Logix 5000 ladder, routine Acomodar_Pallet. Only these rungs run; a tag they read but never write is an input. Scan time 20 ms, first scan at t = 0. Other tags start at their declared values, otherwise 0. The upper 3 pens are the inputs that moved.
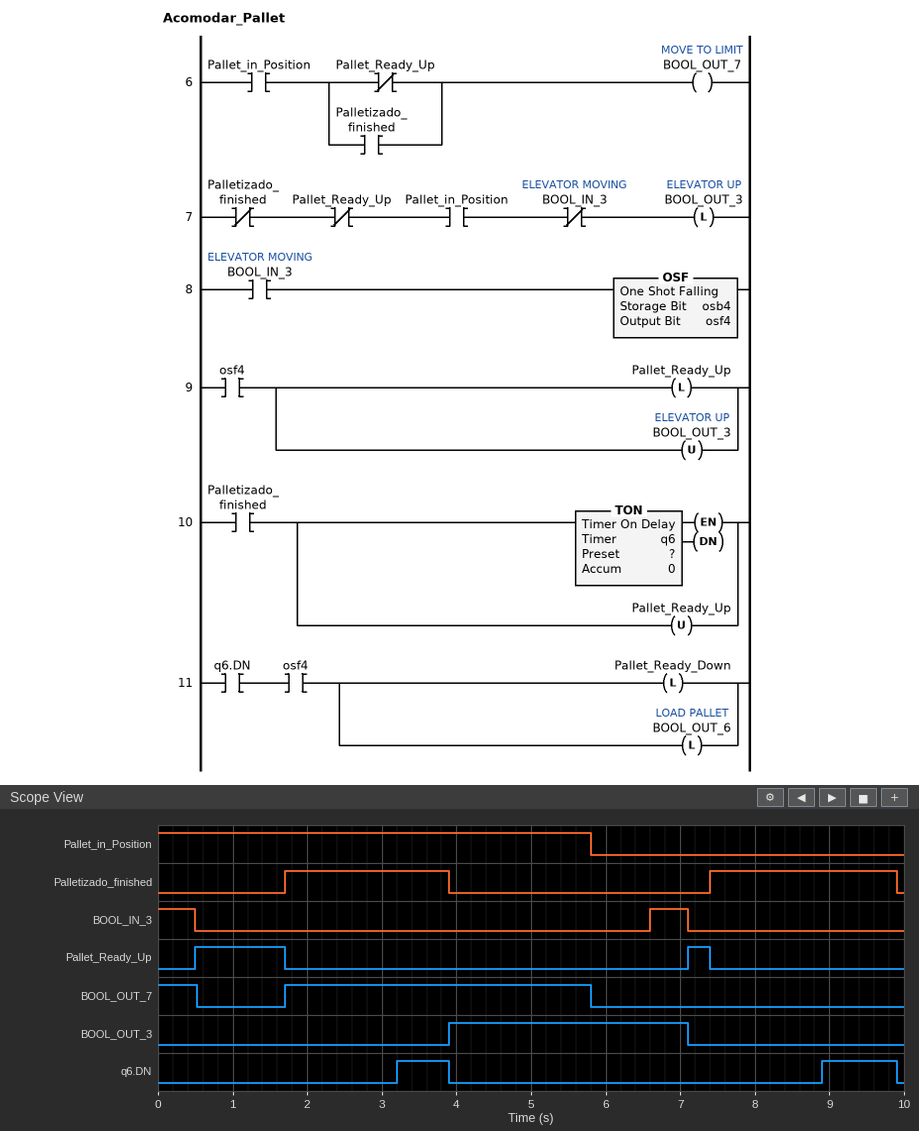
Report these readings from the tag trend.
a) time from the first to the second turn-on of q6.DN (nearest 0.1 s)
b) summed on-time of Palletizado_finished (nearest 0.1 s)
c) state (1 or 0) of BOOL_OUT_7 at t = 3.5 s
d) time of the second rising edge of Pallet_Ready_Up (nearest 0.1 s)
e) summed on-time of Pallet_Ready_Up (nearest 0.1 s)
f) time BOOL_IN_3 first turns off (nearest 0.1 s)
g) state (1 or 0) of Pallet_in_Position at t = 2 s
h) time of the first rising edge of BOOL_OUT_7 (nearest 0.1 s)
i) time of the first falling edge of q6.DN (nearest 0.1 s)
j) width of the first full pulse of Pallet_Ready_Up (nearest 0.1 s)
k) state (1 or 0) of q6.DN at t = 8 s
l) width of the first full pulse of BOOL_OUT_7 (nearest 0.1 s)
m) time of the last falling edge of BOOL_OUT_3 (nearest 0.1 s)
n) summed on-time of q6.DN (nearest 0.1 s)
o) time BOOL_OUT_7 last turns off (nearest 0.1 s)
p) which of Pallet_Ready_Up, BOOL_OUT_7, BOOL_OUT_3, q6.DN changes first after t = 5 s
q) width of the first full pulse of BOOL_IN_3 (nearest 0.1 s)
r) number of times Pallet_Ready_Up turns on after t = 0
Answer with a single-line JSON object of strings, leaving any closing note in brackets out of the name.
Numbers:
{"time from the first to the second turn-on of q6.DN": "5.7 s", "summed on-time of Palletizado_finished": "4.7 s", "state (1 or 0) of BOOL_OUT_7 at t = 3.5 s": "1", "time of the second rising edge of Pallet_Ready_Up": "7.1 s", "summed on-time of Pallet_Ready_Up": "1.5 s", "time BOOL_IN_3 first turns off": "0.5 s", "state (1 or 0) of Pallet_in_Position at t = 2 s": "1", "time of the first rising edge of BOOL_OUT_7": "1.7 s", "time of the first falling edge of q6.DN": "3.9 s", "width of the first full pulse of Pallet_Ready_Up": "1.2 s", "state (1 or 0) of q6.DN at t = 8 s": "0", "width of the first full pulse of BOOL_OUT_7": "4.1 s", "time of the last falling edge of BOOL_OUT_3": "7.1 s", "summed on-time of q6.DN": "1.7 s", "time BOOL_OUT_7 last turns off": "5.8 s", "which of Pallet_Ready_Up, BOOL_OUT_7, BOOL_OUT_3, q6.DN changes first after t = 5 s": "BOOL_OUT_7", "width of the first full pulse of BOOL_IN_3": "0.5 s", "number of times Pallet_Ready_Up turns on after t = 0": "2"}
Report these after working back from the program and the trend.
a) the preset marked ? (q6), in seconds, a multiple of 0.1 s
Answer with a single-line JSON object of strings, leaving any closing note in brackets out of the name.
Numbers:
{"the preset marked ? (q6), in seconds, a multiple of 0.1 s": "1.5 s"}
